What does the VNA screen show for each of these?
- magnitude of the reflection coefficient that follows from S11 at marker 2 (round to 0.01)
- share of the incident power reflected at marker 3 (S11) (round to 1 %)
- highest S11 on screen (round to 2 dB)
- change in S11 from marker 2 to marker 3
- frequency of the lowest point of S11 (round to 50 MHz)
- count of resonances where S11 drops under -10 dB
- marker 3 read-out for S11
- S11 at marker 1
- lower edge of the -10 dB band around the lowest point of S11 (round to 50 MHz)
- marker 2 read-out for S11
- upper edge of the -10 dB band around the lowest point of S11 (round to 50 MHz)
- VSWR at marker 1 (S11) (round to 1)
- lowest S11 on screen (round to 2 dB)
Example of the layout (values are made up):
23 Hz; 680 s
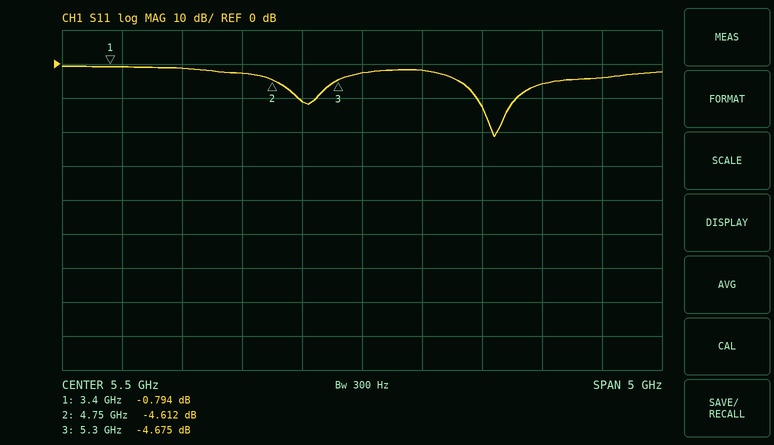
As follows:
0.59; 34 %; 0 dB; -0.063 dB; 6.60 GHz; 2; -4.675 dB; -0.794 dB; 6.45 GHz; -4.612 dB; 6.80 GHz; 22; -22 dB
